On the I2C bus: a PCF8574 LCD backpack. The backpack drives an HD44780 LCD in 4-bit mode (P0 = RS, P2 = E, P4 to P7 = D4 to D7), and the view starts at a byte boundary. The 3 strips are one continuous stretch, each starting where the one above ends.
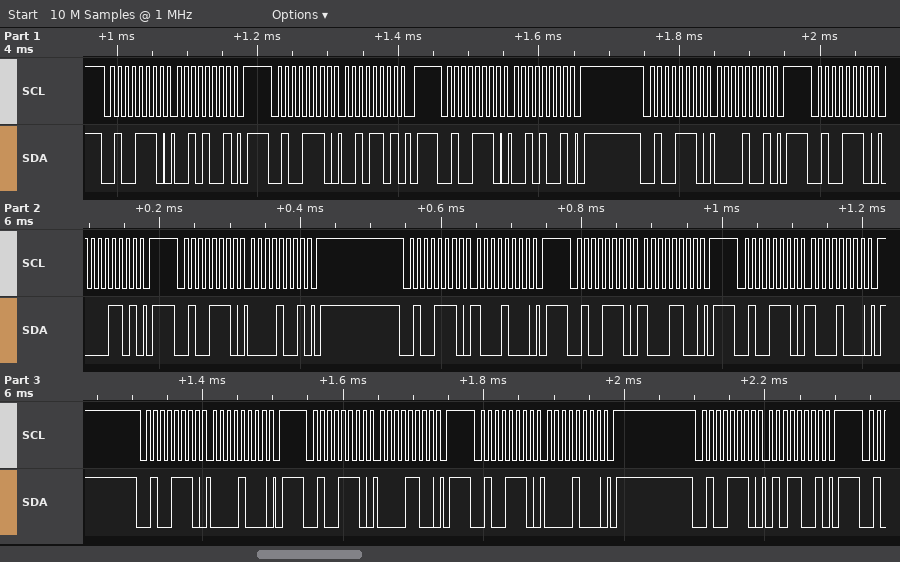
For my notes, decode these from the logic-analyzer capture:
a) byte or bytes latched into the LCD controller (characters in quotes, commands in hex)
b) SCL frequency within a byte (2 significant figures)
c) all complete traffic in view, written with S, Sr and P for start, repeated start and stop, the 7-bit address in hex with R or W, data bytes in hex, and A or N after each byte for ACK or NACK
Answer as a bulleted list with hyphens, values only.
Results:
- ' ' 0x80
- 100 kHz
- S 27W A 29 A P S 27W A 2D A P S 27W A 29 A P S 27W A 09 A P S 27W A 0D A P S 27W A 09 A P S 27W A 88 A P S 27W A 8C A P S 27W A 88 A P S 27W A 08 A P S 27W A 0C A P S 27W A 08 A P S 27W A 59 A P
